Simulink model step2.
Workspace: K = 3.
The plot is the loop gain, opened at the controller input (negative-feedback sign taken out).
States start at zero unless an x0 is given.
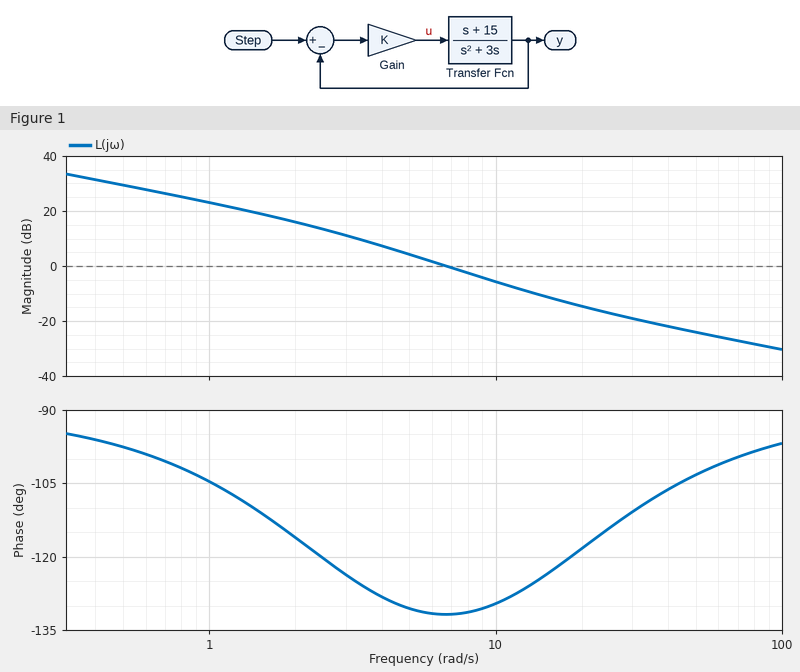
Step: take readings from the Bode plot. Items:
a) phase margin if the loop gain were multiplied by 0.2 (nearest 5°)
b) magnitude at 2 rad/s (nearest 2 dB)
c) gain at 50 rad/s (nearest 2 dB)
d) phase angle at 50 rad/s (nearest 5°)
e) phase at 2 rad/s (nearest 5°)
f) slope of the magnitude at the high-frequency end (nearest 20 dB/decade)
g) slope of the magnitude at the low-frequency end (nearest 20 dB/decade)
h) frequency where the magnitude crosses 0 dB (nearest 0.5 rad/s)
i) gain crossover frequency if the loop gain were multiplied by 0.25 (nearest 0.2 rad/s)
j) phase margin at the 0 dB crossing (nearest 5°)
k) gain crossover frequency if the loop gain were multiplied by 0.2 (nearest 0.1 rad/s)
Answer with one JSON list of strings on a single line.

["60°", "16 dB", "-24 dB", "-105°", "-115°", "-20 dB/decade", "-20 dB/decade", "6.5 rad/s", "2.8 rad/s", "50°", "2.4 rad/s"]
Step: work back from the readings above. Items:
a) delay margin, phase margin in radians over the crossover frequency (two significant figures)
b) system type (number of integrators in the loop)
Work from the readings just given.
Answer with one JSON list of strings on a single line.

["0.13 s", "1"]
